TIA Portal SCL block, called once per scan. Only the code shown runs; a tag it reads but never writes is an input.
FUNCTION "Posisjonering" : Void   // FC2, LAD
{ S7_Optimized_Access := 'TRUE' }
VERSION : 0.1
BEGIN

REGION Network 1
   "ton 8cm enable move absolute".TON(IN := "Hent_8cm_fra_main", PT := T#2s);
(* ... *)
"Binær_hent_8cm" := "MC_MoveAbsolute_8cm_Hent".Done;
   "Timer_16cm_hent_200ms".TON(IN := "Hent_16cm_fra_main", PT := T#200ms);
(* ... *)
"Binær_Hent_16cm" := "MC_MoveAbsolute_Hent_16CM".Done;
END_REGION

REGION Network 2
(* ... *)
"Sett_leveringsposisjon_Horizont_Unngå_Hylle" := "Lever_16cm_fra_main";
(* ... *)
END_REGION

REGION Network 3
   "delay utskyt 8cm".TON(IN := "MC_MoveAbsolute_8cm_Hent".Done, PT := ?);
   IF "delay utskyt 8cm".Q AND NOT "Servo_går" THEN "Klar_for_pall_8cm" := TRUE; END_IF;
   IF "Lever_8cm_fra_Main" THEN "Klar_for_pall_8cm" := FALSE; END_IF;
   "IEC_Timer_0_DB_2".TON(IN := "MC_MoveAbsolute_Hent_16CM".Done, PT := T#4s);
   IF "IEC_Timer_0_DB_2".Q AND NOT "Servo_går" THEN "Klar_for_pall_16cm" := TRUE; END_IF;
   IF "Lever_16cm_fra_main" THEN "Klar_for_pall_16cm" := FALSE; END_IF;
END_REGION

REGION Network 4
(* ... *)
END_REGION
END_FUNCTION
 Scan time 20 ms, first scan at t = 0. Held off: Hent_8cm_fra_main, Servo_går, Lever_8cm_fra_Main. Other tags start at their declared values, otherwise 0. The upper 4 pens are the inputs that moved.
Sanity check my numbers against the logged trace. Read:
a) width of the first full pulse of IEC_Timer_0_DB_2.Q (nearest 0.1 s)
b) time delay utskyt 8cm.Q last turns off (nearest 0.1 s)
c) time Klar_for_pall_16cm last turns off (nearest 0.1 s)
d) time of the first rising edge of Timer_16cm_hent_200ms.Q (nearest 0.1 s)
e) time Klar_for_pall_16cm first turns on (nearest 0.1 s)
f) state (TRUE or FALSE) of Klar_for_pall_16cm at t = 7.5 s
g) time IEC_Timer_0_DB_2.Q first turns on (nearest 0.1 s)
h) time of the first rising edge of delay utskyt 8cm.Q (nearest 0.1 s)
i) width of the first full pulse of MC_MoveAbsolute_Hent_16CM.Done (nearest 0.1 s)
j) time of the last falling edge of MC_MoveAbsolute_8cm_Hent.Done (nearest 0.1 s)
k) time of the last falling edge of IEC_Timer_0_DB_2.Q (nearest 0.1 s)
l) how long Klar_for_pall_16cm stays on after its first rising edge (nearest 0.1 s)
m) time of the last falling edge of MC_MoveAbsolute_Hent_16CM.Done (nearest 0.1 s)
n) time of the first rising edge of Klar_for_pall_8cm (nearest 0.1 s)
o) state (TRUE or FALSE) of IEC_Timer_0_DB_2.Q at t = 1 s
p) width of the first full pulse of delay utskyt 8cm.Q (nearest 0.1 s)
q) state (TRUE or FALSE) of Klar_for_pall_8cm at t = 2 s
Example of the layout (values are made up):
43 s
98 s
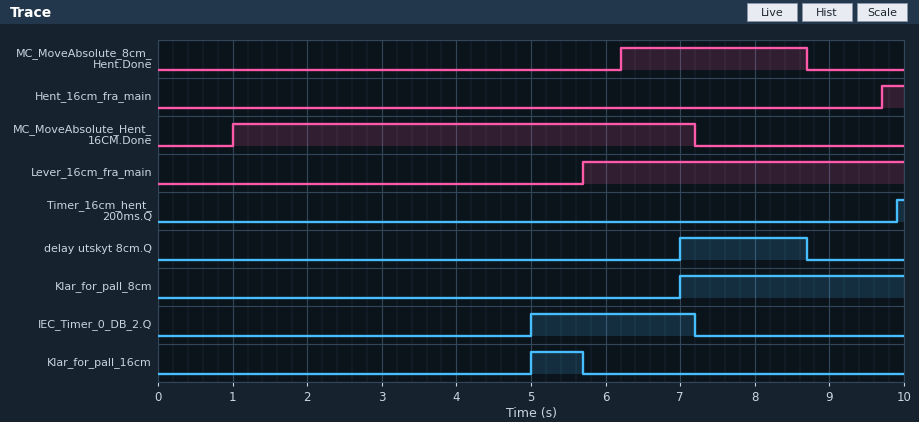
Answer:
2.2 s
8.7 s
5.7 s
9.9 s
5.0 s
FALSE
5.0 s
7.0 s
6.2 s
8.7 s
7.2 s
0.7 s
7.2 s
7.0 s
FALSE
1.7 s
FALSE
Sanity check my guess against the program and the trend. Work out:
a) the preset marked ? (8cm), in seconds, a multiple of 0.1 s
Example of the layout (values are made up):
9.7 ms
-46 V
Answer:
0.8 s
